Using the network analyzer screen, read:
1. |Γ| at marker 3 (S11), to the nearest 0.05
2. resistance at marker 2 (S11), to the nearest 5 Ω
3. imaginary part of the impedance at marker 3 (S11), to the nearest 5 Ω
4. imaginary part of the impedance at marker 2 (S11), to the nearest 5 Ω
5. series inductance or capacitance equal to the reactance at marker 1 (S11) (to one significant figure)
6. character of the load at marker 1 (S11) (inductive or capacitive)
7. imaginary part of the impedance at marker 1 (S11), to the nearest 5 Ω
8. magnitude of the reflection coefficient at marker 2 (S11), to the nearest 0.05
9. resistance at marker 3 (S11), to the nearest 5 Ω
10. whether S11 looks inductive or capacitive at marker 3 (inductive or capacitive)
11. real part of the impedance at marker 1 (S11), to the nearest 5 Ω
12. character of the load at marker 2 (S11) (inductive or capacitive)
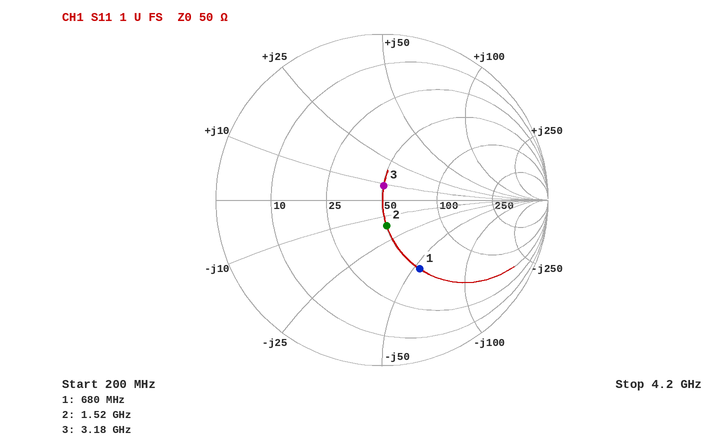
0.10
50 Ω
+10 Ω
-15 Ω
4 pF
capacitive
-55 Ω
0.15
50 Ω
inductive
50 Ω
capacitive
